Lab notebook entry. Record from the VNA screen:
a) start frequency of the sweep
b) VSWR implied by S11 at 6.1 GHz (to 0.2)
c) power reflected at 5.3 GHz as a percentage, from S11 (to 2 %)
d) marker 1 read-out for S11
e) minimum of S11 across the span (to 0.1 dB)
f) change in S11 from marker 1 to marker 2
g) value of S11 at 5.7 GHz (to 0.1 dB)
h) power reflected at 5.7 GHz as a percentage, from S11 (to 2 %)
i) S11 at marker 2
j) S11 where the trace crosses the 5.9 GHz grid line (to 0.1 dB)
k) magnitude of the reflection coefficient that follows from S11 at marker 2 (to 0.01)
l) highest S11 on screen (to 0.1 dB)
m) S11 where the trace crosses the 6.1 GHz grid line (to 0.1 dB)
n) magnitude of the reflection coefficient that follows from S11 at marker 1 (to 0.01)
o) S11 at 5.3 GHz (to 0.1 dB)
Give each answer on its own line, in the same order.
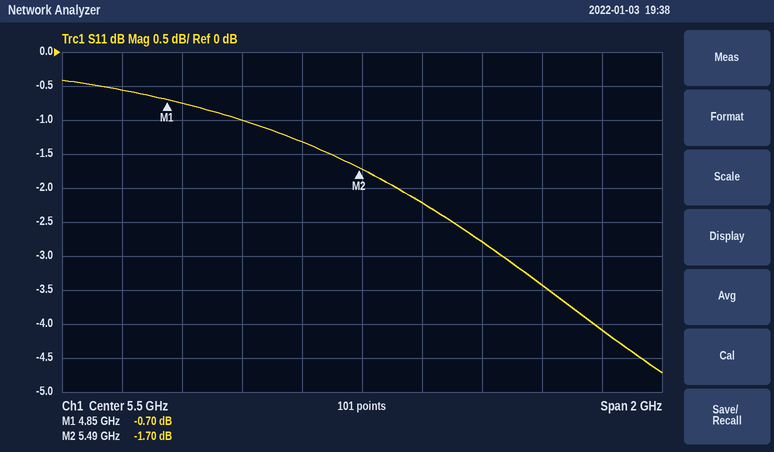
4.5 GHz
5.2
74 %
-0.70 dB
-4.7 dB
-1.00 dB
-2.2 dB
60 %
-1.70 dB
-2.8 dB
0.82
-0.4 dB
-3.4 dB
0.92
-1.3 dB
